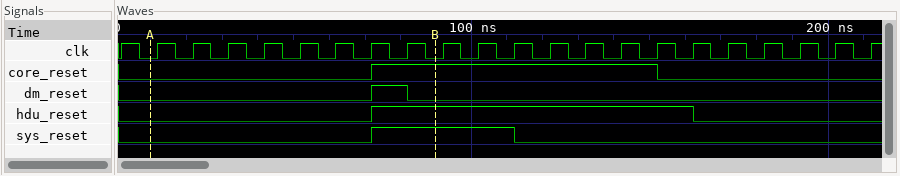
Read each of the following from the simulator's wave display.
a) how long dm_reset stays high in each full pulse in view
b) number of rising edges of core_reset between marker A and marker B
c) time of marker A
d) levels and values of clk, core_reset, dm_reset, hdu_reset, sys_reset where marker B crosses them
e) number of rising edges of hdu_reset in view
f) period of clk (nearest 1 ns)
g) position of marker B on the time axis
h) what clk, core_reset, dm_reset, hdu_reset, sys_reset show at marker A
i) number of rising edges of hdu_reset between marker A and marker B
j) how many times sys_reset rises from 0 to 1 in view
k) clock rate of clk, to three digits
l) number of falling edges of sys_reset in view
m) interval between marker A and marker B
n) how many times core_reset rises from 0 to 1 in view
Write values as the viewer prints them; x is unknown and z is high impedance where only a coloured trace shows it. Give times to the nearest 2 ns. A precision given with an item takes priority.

10 ns
1
10 ns
clk=0, core_reset=1, dm_reset=0, hdu_reset=1, sys_reset=1
1
10 ns
90 ns
clk=0, core_reset=0, dm_reset=0, hdu_reset=0, sys_reset=0
1
1
100 MHz
1
80 ns
1
